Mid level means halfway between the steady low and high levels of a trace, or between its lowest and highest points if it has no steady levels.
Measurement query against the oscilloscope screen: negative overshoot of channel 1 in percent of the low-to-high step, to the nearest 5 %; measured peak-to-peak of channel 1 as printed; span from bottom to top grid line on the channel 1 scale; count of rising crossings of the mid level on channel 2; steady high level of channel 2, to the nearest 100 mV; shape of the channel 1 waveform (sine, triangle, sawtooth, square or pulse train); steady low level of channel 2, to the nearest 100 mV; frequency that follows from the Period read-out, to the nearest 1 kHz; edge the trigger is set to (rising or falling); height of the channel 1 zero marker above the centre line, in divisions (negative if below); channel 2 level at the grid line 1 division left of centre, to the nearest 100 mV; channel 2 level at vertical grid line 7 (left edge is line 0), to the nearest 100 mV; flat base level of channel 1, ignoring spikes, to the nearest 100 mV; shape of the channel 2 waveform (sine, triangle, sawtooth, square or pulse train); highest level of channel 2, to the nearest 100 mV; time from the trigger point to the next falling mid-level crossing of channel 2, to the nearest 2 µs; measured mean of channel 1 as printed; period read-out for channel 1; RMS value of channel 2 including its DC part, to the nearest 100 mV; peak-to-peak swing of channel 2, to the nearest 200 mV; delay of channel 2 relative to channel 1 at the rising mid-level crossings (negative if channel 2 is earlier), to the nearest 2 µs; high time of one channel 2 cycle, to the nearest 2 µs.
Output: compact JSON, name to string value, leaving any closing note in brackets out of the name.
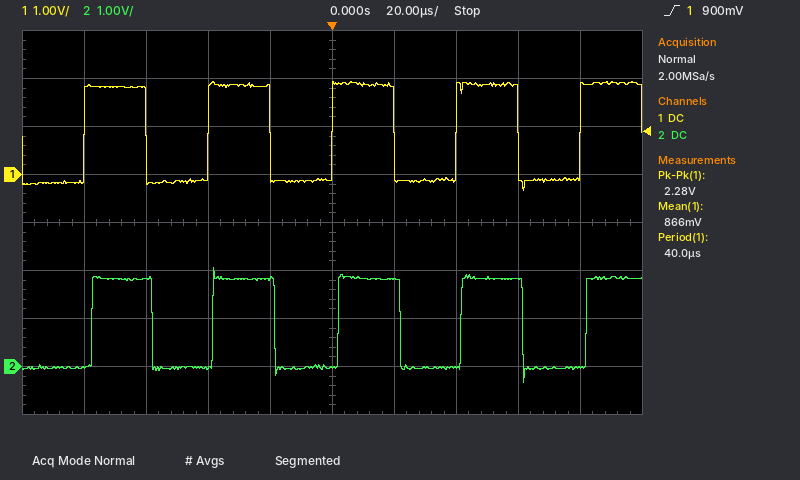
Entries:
{"negative overshoot of channel 1 in percent of the low-to-high step, to the nearest 5 %": "10 %", "measured peak-to-peak of channel 1 as printed": "2.28 V", "span from bottom to top grid line on the channel 1 scale": "8 V", "count of rising crossings of the mid level on channel 2": "5", "steady high level of channel 2, to the nearest 100 mV": "1.8 V", "shape of the channel 1 waveform": "square", "steady low level of channel 2, to the nearest 100 mV": "0.0 V", "frequency that follows from the Period read-out, to the nearest 1 kHz": "25 kHz", "edge the trigger is set to": "rising", "height of the channel 1 zero marker above the centre line, in divisions": "+1.0 div", "channel 2 level at the grid line 1 division left of centre, to the nearest 100 mV": "1.8 V", "channel 2 level at vertical grid line 7 (left edge is line 0), to the nearest 100 mV": "0.0 V", "flat base level of channel 1, ignoring spikes, to the nearest 100 mV": "-100 mV", "shape of the channel 2 waveform": "square", "highest level of channel 2, to the nearest 100 mV": "2.1 V", "time from the trigger point to the next falling mid-level crossing of channel 2, to the nearest 2 µs": "22 µs", "measured mean of channel 1 as printed": "866 mV", "period read-out for channel 1": "40.0 µs", "RMS value of channel 2 including its DC part, to the nearest 100 mV": "1.3 V", "peak-to-peak swing of channel 2, to the nearest 200 mV": "2.4 V", "delay of channel 2 relative to channel 1 at the rising mid-level crossings (negative if channel 2 is earlier), to the nearest 2 µs": "+2 µs", "high time of one channel 2 cycle, to the nearest 2 µs": "20 µs"}
